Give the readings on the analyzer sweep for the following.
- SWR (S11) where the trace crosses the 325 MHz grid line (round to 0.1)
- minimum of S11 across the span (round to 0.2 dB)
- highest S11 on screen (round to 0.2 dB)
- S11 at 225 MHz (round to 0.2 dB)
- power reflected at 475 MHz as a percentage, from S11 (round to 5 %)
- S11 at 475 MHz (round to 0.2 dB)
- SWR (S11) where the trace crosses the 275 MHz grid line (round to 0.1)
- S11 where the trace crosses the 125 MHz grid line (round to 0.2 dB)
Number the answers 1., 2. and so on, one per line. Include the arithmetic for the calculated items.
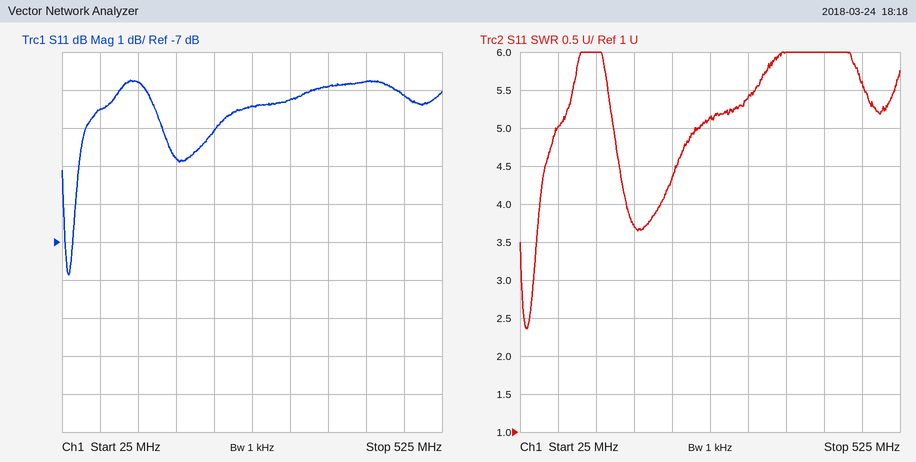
1. 5.4
2. -7.8 dB
3. -2.8 dB
4. -4.0 dB
5. 10^(-3.2/10) ≈ 47.9 %, so 50 % to the nearest 5 %
6. -3.2 dB
7. 5.1
8. -2.8 dB
